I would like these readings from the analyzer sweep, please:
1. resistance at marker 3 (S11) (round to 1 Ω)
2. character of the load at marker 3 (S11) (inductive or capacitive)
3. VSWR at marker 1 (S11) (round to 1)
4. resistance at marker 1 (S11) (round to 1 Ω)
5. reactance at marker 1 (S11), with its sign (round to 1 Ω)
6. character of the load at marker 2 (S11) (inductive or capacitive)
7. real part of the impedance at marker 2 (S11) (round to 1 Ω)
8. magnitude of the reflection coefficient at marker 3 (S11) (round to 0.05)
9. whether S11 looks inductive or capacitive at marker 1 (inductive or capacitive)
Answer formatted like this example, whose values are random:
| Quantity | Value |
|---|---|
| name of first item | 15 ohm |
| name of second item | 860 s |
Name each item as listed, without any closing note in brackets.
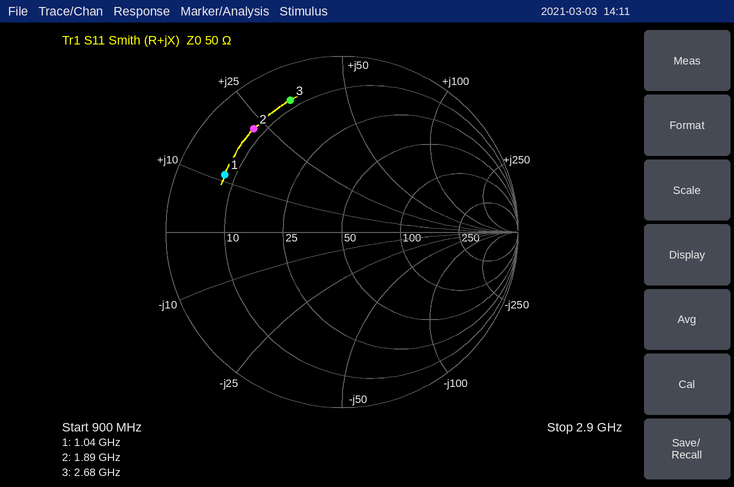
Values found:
| Quantity | Value |
|---|---|
| resistance at marker 3 (S11) | 8 Ω |
| character of the load at marker 3 (S11) | inductive |
| VSWR at marker 1 (S11) | 7 |
| resistance at marker 1 (S11) | 8 Ω |
| reactance at marker 1 (S11), with its sign | +11 Ω |
| character of the load at marker 2 (S11) | inductive |
| real part of the impedance at marker 2 (S11) | 8 Ω |
| magnitude of the reflection coefficient at marker 3 (S11) | 0.80 |
| whether S11 looks inductive or capacitive at marker 1 | inductive |
